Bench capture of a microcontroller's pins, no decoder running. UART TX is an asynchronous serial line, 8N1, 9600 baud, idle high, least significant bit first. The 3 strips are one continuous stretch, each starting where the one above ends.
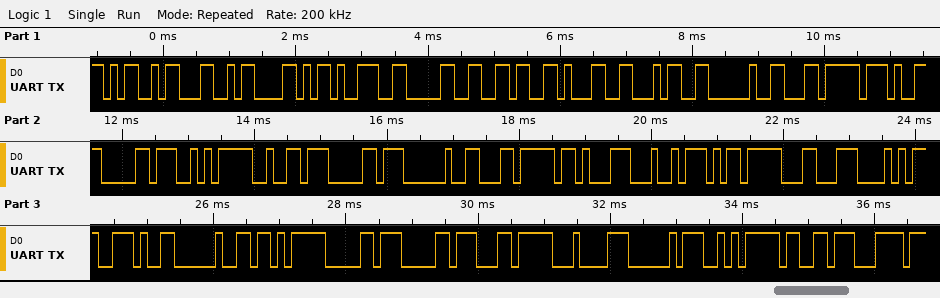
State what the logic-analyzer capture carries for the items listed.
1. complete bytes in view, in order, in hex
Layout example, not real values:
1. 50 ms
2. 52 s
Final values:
1. 4D 4C 58 39 30 36 31 34 20 EC 97 B0 EA B2 B0 20 EC 8B A4 ED 8C A8 2E 20 EB B0 B0 EC 84 A0 EA B3 BC
